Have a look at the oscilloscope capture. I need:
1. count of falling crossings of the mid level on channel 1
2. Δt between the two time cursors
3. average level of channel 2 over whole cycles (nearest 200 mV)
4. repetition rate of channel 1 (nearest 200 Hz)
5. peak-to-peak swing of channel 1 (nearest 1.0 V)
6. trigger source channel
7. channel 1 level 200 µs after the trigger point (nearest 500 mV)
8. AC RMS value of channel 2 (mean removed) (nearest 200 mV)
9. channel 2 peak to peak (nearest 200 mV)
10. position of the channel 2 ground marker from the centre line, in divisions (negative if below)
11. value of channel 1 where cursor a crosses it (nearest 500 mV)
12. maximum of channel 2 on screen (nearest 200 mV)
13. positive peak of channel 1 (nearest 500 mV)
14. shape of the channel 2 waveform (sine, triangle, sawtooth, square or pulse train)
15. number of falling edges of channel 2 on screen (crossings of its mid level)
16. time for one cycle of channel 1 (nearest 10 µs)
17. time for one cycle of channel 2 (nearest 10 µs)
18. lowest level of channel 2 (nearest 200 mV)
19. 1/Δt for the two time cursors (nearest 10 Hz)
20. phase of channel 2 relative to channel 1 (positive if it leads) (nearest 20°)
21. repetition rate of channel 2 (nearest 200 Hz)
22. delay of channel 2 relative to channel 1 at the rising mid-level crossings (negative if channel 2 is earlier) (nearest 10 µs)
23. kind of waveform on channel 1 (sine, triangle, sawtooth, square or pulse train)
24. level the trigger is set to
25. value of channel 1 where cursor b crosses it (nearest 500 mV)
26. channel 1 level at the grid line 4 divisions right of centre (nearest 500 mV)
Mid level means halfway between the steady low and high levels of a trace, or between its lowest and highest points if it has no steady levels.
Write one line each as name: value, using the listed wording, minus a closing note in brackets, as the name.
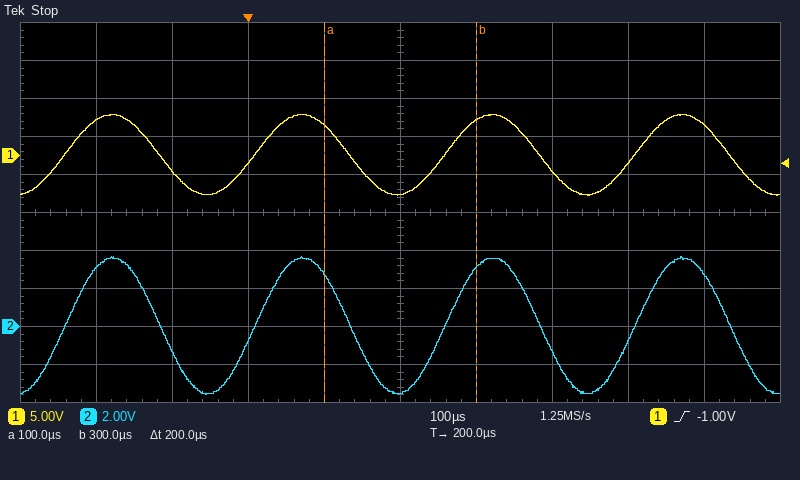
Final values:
count of falling crossings of the mid level on channel 1: 4
Δt between the two time cursors: 200 µs
average level of channel 2 over whole cycles: 0.0 V
repetition rate of channel 1: 4.0 kHz
peak-to-peak swing of channel 1: 11.0 V
trigger source channel: channel 1
channel 1 level 200 µs after the trigger point: -5.0 V
AC RMS value of channel 2 (mean removed): 2.6 V
channel 2 peak to peak: 7.2 V
position of the channel 2 ground marker from the centre line, in divisions: -3.0 div
value of channel 1 where cursor a crosses it: 4.0 V
maximum of channel 2 on screen: 3.6 V
positive peak of channel 1: 5.5 V
shape of the channel 2 waveform: sine
number of falling edges of channel 2 on screen: 4
time for one cycle of channel 1: 250 µs
time for one cycle of channel 2: 250 µs
lowest level of channel 2: -3.6 V
1/Δt for the two time cursors: 5.00 kHz
phase of channel 2 relative to channel 1 (positive if it leads): 0°
repetition rate of channel 2: 4.0 kHz
delay of channel 2 relative to channel 1 at the rising mid-level crossings (negative if channel 2 is earlier): 0 µs
kind of waveform on channel 1: sine
level the trigger is set to: -1.00 V
value of channel 1 where cursor b crosses it: 4.5 V
channel 1 level at the grid line 4 divisions right of centre: 4.0 V
